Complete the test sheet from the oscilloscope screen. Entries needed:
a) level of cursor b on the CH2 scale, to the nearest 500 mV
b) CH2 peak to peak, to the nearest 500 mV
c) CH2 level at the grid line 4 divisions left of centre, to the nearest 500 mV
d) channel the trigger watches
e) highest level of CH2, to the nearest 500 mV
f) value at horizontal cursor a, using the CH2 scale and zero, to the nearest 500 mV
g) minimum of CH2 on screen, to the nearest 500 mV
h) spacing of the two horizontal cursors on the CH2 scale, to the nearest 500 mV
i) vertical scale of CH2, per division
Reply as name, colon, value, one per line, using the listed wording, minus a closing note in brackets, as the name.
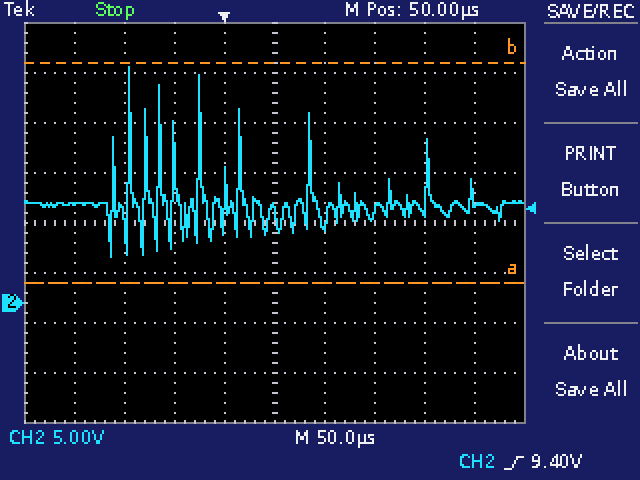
level of cursor b on the CH2 scale, to the nearest 500 mV: 24.0 V
CH2 peak to peak, to the nearest 500 mV: 19.0 V
CH2 level at the grid line 4 divisions left of centre, to the nearest 500 mV: 10.0 V
channel the trigger watches: CH2
highest level of CH2, to the nearest 500 mV: 23.5 V
value at horizontal cursor a, using the CH2 scale and zero, to the nearest 500 mV: 2.0 V
minimum of CH2 on screen, to the nearest 500 mV: 4.5 V
spacing of the two horizontal cursors on the CH2 scale, to the nearest 500 mV: 22.0 V
vertical scale of CH2, per division: 5 V
